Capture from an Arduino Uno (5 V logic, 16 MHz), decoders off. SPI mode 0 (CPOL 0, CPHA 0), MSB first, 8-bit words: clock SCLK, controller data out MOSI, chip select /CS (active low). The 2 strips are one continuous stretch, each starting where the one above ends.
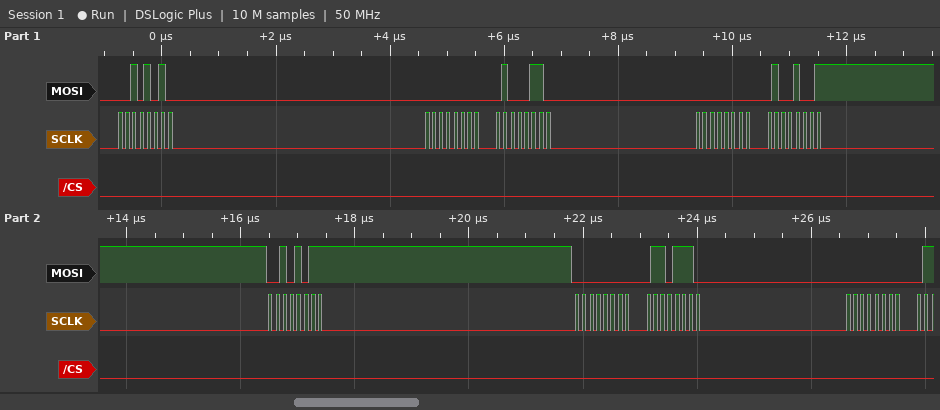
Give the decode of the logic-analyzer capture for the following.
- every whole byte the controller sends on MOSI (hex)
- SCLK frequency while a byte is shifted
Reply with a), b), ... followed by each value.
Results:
a) 2A 00 46 00 49 2B 00 6E 00
b) 8 MHz
